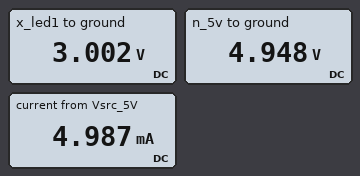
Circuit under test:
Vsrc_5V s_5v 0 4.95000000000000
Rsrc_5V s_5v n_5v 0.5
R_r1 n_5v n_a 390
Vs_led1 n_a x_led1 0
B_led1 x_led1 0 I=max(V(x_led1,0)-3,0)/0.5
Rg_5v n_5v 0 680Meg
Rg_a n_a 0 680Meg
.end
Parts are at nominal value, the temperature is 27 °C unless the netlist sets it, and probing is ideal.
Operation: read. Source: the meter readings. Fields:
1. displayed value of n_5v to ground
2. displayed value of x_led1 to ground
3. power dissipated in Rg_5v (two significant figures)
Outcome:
4.948 V
3.002 V
36 nW
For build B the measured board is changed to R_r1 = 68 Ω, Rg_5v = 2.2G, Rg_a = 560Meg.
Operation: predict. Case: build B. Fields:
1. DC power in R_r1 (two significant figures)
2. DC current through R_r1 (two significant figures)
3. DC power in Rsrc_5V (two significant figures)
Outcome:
54 mW
28 mA
400 µW
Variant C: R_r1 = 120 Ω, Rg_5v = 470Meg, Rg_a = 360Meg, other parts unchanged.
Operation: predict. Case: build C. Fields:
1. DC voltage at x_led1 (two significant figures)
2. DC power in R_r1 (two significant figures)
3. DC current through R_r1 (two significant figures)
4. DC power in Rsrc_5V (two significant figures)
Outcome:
3.0 V
31 mW
16 mA
130 µW
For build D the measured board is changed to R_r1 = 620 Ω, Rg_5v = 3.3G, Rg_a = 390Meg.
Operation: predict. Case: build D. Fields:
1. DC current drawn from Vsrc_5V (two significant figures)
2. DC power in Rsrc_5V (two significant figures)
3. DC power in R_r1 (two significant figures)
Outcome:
3.1 mA
4.9 µW
6.1 mW
